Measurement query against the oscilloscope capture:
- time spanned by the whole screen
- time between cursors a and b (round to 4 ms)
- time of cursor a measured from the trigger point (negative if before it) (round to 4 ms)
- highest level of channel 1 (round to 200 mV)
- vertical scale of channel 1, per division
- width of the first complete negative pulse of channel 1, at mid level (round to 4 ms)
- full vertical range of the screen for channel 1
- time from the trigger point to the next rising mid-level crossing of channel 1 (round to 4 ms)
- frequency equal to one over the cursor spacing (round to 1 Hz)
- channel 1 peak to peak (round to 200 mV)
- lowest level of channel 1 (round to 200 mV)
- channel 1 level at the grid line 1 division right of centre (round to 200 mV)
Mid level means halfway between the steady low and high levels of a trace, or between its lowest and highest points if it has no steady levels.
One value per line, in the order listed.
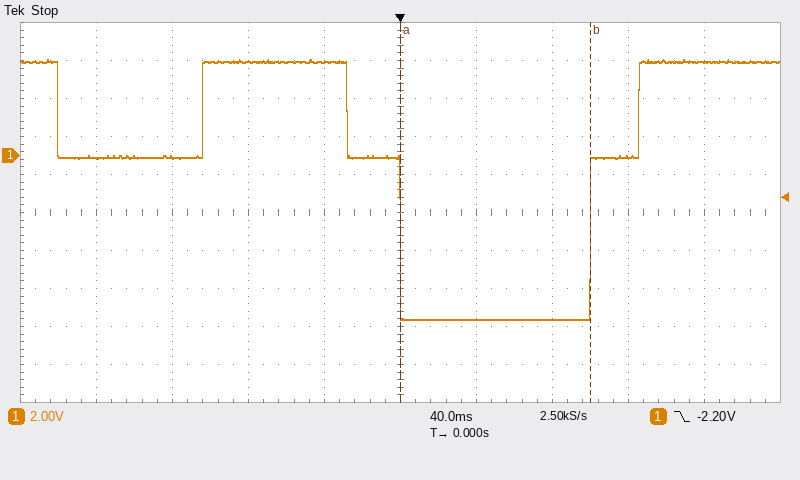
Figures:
400 ms
100 ms
0 ms
5.0 V
2 V
100 ms
20 V
100 ms
10 Hz
13.6 V
-8.6 V
-8.6 V
